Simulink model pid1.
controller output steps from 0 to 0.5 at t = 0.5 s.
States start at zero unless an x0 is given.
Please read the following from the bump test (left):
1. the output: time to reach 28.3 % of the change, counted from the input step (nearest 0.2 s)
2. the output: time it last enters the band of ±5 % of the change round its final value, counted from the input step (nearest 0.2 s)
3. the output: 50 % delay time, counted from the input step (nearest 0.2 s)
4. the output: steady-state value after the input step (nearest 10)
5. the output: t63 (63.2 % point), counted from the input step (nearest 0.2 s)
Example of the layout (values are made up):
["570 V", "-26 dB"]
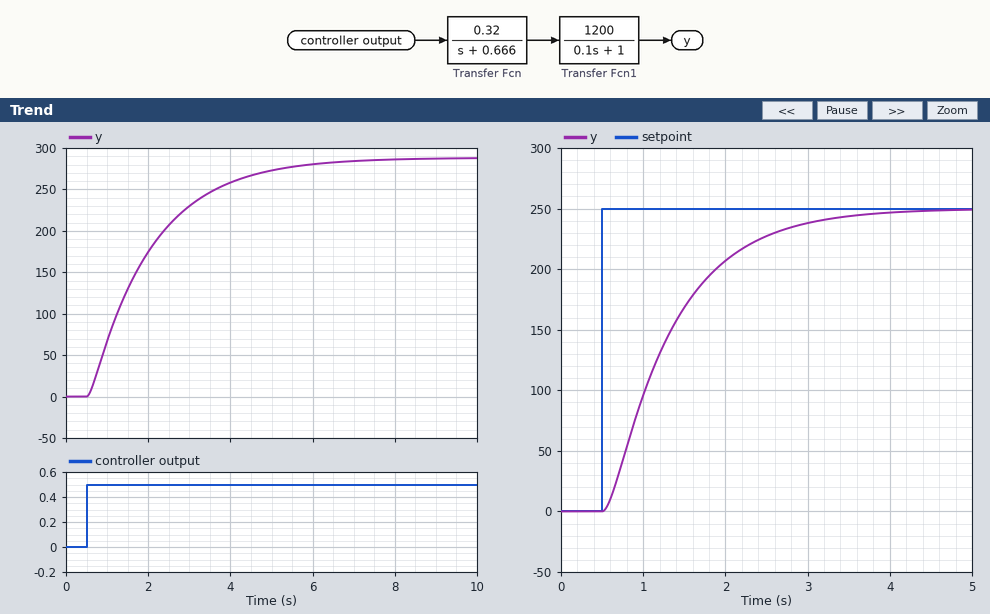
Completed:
["0.6 s", "4.6 s", "1.2 s", "290", "1.6 s"]
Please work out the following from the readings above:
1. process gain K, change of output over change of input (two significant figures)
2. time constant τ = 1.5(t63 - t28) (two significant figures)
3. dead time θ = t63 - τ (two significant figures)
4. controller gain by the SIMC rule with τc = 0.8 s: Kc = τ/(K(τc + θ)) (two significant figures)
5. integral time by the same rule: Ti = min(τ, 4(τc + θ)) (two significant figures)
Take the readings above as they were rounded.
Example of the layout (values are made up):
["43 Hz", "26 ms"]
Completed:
["580", "1.5 s", "0.10 s", "0.0029", "1.5 s"]
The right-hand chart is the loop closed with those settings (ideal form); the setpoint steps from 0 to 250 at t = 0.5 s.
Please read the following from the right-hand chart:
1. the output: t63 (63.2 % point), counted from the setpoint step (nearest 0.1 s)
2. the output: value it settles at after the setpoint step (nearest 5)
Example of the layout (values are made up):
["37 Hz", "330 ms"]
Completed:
["0.9 s", "250"]
